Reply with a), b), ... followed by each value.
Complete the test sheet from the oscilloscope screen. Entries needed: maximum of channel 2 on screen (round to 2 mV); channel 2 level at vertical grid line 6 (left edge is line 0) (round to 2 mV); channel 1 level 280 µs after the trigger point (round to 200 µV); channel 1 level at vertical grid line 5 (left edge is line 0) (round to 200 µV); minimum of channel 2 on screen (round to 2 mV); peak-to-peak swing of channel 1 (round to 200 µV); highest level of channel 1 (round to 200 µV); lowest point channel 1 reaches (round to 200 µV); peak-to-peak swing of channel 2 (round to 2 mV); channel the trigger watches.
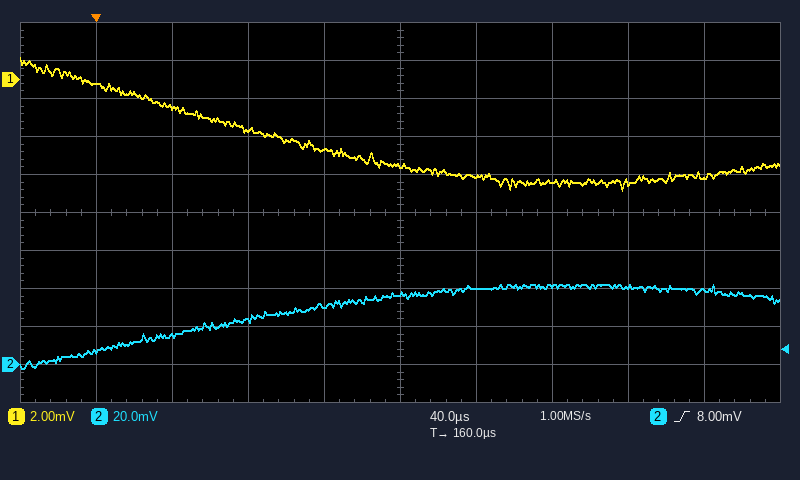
a) 42 mV
b) 40 mV
c) -5.4 mV
d) -4.6 mV
e) -2 mV
f) 7.0 mV
g) 1.2 mV
h) -5.8 mV
i) 44 mV
j) channel 2
